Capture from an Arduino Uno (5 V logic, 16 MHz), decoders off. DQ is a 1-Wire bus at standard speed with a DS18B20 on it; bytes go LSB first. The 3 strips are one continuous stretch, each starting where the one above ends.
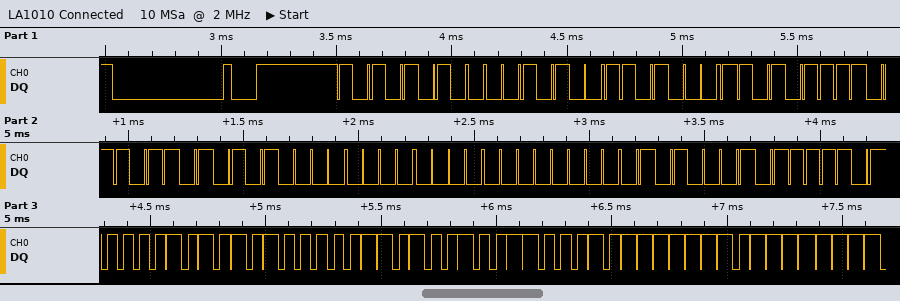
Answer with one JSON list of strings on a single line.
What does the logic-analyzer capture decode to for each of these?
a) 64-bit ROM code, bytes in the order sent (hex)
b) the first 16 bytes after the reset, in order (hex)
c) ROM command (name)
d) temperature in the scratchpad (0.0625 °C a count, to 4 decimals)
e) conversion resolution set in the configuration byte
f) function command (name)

["28 8B F5 B6 0A 00 00 8A", "55 28 8B F5 B6 0A 00 00 8A BE 50 05 4B 46 7F FF", "Match ROM", "85.0000 °C", "12 bits", "Read Scratchpad"]
